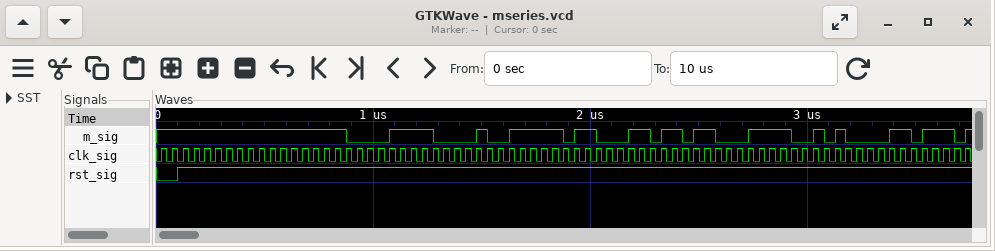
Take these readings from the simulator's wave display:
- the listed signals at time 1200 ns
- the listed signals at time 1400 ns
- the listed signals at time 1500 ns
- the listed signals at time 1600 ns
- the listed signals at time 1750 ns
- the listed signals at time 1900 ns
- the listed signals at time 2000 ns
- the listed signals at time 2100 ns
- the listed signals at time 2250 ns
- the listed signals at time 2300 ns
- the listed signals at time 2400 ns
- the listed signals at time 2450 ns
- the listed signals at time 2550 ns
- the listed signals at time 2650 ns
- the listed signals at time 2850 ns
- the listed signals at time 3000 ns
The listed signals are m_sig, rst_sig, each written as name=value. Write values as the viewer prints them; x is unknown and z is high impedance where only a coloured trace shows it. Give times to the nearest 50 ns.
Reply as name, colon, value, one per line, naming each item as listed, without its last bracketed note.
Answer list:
the listed signals at time 1200 ns: m_sig=1, rst_sig=1
the listed signals at time 1400 ns: m_sig=0, rst_sig=1
the listed signals at time 1500 ns: m_sig=1, rst_sig=1
the listed signals at time 1600 ns: m_sig=0, rst_sig=1
the listed signals at time 1750 ns: m_sig=1, rst_sig=1
the listed signals at time 1900 ns: m_sig=0, rst_sig=1
the listed signals at time 2000 ns: m_sig=1, rst_sig=1
the listed signals at time 2100 ns: m_sig=0, rst_sig=1
the listed signals at time 2250 ns: m_sig=1, rst_sig=1
the listed signals at time 2300 ns: m_sig=0, rst_sig=1
the listed signals at time 2400 ns: m_sig=1, rst_sig=1
the listed signals at time 2450 ns: m_sig=0, rst_sig=1
the listed signals at time 2550 ns: m_sig=1, rst_sig=1
the listed signals at time 2650 ns: m_sig=0, rst_sig=1
the listed signals at time 2850 ns: m_sig=1, rst_sig=1
the listed signals at time 3000 ns: m_sig=0, rst_sig=1
